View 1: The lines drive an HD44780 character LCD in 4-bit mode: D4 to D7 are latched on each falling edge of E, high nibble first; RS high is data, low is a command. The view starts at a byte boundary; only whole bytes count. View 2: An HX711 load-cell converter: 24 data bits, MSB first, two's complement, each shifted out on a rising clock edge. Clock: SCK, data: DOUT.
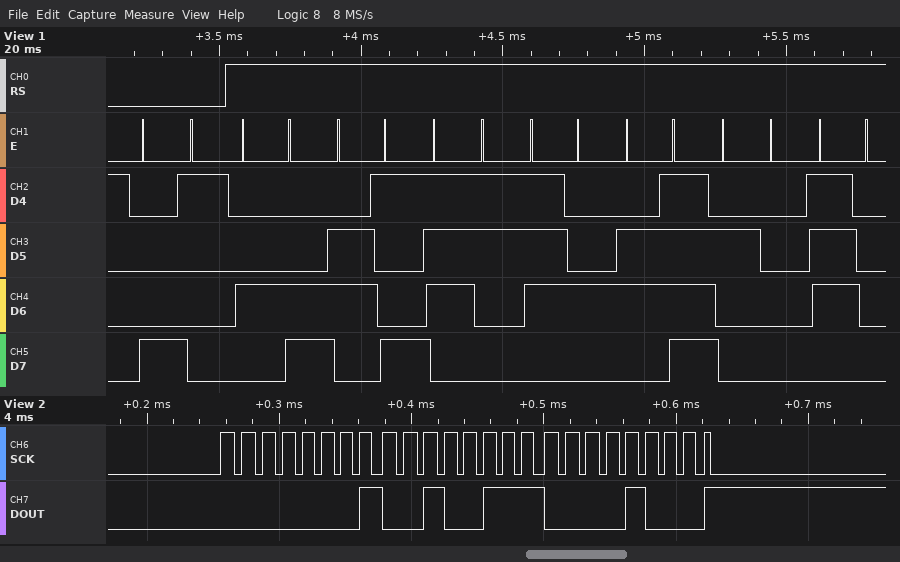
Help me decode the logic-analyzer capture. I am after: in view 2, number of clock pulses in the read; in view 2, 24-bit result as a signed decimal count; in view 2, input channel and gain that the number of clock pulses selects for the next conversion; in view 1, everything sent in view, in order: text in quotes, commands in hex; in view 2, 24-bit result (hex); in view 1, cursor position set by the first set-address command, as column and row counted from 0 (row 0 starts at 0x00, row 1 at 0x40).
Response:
25
75528
channel A, gain 128
0x81 "Listo p"
0x012708
column 1, row 0
